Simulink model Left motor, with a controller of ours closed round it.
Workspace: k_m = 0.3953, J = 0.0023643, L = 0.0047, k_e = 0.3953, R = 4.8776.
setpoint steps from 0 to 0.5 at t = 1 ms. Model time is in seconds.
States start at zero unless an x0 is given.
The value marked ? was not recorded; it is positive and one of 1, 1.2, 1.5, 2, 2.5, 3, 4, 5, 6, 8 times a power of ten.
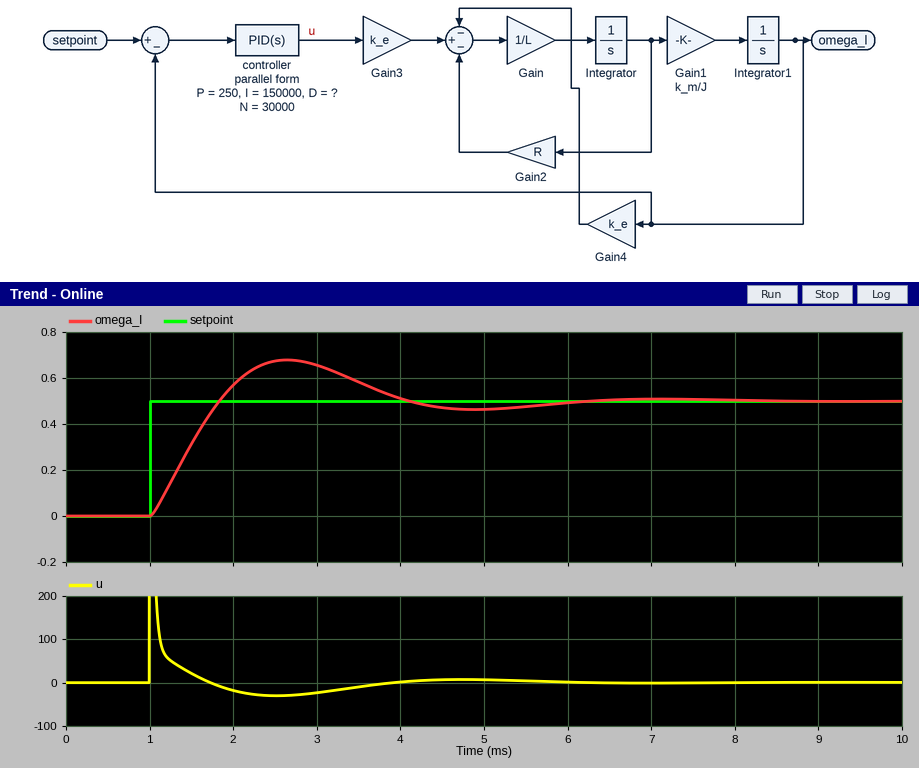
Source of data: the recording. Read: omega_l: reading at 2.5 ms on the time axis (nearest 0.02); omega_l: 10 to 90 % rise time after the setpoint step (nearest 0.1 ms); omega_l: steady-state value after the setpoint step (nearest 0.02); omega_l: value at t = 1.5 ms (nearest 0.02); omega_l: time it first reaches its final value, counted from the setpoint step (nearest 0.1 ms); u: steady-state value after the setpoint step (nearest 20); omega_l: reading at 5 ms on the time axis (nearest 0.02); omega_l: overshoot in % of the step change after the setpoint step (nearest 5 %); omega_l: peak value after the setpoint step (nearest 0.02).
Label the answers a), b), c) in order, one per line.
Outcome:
a) 0.68
b) 0.6 ms
c) 0.50
d) 0.32
e) 0.8 ms
f) 0
g) 0.46
h) 35 %
i) 0.68
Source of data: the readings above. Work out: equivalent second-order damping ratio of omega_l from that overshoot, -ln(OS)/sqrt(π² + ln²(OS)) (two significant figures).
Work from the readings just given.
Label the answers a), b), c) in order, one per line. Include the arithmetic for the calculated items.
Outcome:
a) ln(0.35) = -1.050; 1.050 / sqrt(9.870 + 1.102) = 0.32
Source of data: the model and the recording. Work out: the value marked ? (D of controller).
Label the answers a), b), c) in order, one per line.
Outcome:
a) 0.08
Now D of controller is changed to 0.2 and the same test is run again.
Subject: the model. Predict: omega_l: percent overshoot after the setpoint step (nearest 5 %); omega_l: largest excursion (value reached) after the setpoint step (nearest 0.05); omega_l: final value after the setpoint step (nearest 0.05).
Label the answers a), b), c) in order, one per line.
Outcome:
a) 15 %
b) 0.55
c) 0.50
